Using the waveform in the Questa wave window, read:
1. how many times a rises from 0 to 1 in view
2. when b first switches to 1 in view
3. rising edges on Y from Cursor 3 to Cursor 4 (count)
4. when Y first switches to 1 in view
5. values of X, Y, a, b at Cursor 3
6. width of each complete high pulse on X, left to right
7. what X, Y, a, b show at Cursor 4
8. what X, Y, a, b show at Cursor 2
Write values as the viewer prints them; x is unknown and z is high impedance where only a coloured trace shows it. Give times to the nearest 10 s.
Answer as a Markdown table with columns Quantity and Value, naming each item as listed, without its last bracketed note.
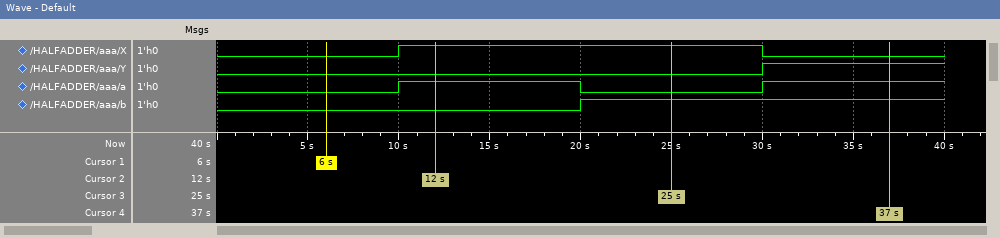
| Quantity | Value |
|---|---|
| how many times a rises from 0 to 1 in view | 2 |
| when b first switches to 1 in view | 20 s |
| rising edges on Y from Cursor 3 to Cursor 4 | 1 |
| when Y first switches to 1 in view | 30 s |
| values of X, Y, a, b at Cursor 3 | X=1, Y=0, a=0, b=1 |
| width of each complete high pulse on X, left to right | 20 s |
| what X, Y, a, b show at Cursor 4 | X=0, Y=1, a=1, b=1 |
| what X, Y, a, b show at Cursor 2 | X=1, Y=0, a=1, b=0 |
